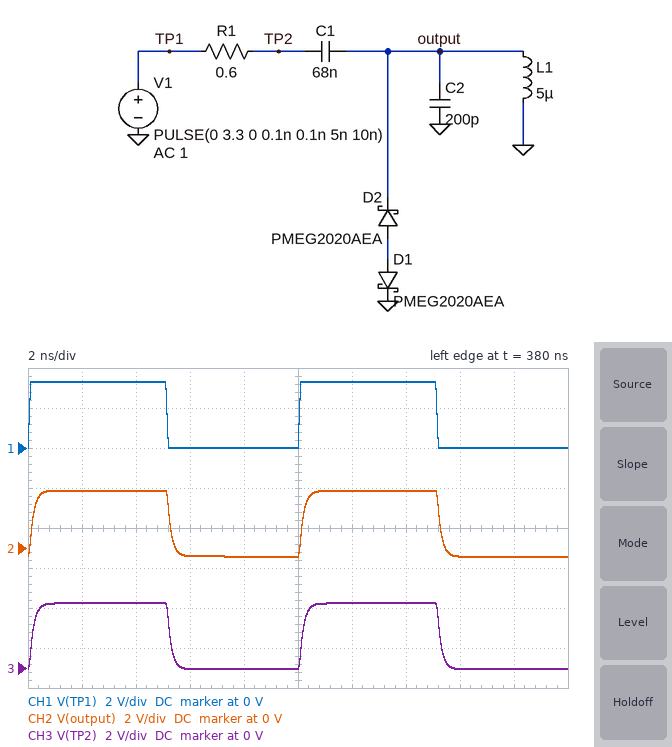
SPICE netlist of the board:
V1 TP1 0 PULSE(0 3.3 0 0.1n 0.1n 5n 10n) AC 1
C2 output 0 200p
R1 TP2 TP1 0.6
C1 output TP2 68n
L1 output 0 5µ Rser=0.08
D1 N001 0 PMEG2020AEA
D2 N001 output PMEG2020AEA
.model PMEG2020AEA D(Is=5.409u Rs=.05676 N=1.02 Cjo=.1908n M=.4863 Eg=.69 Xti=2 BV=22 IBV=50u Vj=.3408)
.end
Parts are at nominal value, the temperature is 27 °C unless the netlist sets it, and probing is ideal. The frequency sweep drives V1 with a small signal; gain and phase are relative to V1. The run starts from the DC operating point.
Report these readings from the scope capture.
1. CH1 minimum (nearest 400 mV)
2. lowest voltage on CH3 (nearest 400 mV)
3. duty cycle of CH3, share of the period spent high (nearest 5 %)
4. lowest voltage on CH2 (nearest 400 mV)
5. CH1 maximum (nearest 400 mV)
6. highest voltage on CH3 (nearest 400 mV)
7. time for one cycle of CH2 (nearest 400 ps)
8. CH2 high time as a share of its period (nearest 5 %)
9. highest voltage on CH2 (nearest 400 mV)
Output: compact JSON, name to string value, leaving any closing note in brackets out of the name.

{"CH1 minimum": "0 V", "lowest voltage on CH3": "0 V", "duty cycle of CH3, share of the period spent high": "50 %", "lowest voltage on CH2": "-400 mV", "CH1 maximum": "3.2 V", "highest voltage on CH3": "3.2 V", "time for one cycle of CH2": "10.0 ns", "CH2 high time as a share of its period": "50 %", "highest voltage on CH2": "2.8 V"}
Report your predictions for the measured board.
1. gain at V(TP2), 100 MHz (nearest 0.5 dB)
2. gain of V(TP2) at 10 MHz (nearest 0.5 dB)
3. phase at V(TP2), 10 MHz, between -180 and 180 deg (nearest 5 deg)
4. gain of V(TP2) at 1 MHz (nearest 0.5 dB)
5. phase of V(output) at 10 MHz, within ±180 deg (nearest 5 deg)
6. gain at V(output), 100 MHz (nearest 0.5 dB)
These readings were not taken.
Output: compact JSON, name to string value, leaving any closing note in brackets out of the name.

{"gain at V(TP2), 100 MHz": "0 dB", "gain of V(TP2) at 10 MHz": "0 dB", "phase at V(TP2), 10 MHz, between -180 and 180 deg": "0 deg", "gain of V(TP2) at 1 MHz": "0 dB", "phase of V(output) at 10 MHz, within ±180 deg": "0 deg", "gain at V(output), 100 MHz": "0 dB"}
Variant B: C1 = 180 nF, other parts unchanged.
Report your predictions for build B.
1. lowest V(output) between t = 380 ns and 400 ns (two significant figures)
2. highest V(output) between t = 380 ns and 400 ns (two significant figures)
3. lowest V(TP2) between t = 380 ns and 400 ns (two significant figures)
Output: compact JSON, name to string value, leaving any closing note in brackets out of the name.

{"lowest V(output) between t = 380 ns and 400 ns": "-220 mV", "highest V(output) between t = 380 ns and 400 ns": "3.1 V", "lowest V(TP2) between t = 380 ns and 400 ns": "-76 mV"}
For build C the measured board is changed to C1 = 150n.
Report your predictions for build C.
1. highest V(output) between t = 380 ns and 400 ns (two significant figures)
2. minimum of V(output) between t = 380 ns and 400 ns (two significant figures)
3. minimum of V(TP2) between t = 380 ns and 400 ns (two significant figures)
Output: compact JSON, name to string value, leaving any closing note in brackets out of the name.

{"highest V(output) between t = 380 ns and 400 ns": "3.1 V", "minimum of V(output) between t = 380 ns and 400 ns": "-250 mV", "minimum of V(TP2) between t = 380 ns and 400 ns": "-76 mV"}
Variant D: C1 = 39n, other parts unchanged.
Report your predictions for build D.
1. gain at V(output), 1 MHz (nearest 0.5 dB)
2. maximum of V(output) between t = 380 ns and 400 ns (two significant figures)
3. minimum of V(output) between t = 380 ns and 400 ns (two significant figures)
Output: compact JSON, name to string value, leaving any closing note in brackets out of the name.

{"gain at V(output), 1 MHz": "1.0 dB", "maximum of V(output) between t = 380 ns and 400 ns": "2.6 V", "minimum of V(output) between t = 380 ns and 400 ns": "-700 mV"}
